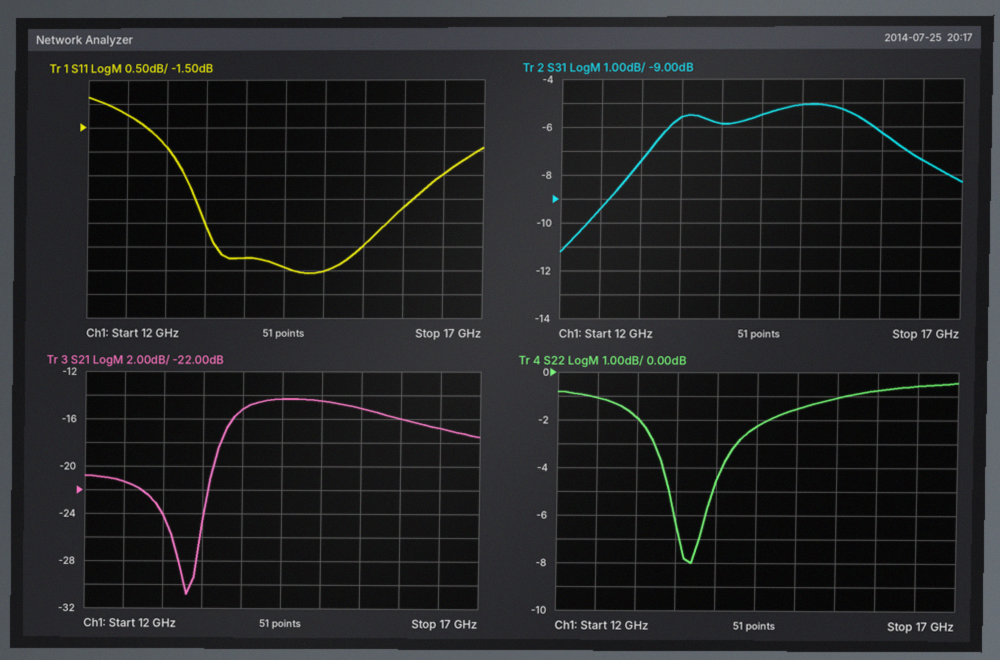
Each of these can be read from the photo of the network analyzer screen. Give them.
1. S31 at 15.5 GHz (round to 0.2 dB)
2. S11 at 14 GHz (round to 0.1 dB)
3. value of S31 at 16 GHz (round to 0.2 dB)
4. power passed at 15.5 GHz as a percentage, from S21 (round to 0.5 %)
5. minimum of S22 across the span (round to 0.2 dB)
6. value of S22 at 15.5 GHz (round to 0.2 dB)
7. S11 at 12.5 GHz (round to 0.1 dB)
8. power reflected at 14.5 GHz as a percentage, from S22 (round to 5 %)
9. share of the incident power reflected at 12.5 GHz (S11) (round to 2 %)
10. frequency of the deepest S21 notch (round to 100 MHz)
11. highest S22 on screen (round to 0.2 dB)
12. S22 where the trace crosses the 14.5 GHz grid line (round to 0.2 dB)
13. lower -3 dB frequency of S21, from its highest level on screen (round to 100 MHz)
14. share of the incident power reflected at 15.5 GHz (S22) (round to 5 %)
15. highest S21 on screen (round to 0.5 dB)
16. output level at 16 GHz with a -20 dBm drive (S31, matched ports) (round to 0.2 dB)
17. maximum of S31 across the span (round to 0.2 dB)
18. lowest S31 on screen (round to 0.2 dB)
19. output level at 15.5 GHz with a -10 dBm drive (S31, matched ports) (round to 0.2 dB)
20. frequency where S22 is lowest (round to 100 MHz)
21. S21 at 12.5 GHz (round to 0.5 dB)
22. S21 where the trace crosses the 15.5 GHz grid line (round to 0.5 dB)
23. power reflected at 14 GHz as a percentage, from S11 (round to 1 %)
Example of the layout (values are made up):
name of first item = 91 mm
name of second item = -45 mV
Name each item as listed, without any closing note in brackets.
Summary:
S31 at 15.5 GHz = -5.2 dB
S11 at 14 GHz = -4.2 dB
value of S31 at 16 GHz = -6.2 dB
power passed at 15.5 GHz as a percentage, from S21 = 3.0 %
minimum of S22 across the span = -8.0 dB
value of S22 at 15.5 GHz = -1.0 dB
S11 at 12.5 GHz = -1.2 dB
power reflected at 14.5 GHz as a percentage, from S22 = 60 %
share of the incident power reflected at 12.5 GHz (S11) = 76 %
frequency of the deepest S21 notch = 13.3 GHz
highest S22 on screen = -0.4 dB
S22 where the trace crosses the 14.5 GHz grid line = -2.2 dB
lower -3 dB frequency of S21, from its highest level on screen = 13.8 GHz
share of the incident power reflected at 15.5 GHz (S22) = 80 %
highest S21 on screen = -14.5 dB
output level at 16 GHz with a -20 dBm drive (S31, matched ports) = -26.2 dBm
maximum of S31 across the span = -5.0 dB
lowest S31 on screen = -11.2 dB
output level at 15.5 GHz with a -10 dBm drive (S31, matched ports) = -15.2 dBm
frequency where S22 is lowest = 13.7 GHz
S21 at 12.5 GHz = -21.5 dB
S21 where the trace crosses the 15.5 GHz grid line = -15.0 dB
power reflected at 14 GHz as a percentage, from S11 = 38 %
